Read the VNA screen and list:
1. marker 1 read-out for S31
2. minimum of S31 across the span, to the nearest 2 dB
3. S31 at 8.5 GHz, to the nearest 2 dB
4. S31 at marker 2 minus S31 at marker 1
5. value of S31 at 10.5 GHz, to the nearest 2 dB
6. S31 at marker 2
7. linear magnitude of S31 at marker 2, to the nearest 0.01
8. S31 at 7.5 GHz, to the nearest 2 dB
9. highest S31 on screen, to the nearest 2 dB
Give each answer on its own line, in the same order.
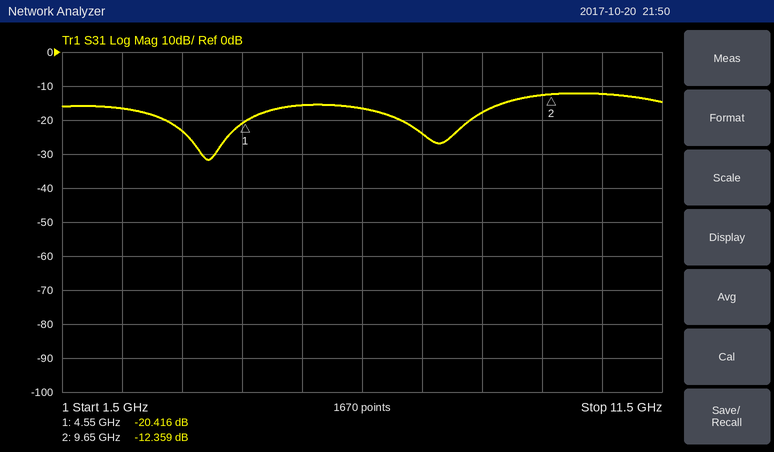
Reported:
-20.416 dB
-32 dB
-18 dB
8.057 dB
-12 dB
-12.359 dB
0.24
-24 dB
-12 dB
